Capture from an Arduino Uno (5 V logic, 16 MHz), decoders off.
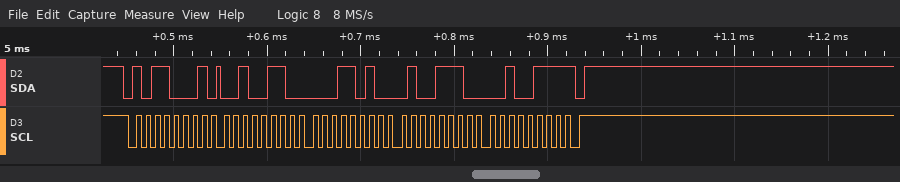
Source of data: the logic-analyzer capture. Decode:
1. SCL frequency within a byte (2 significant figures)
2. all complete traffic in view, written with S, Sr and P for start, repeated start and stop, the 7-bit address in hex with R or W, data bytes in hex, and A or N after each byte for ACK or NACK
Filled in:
100 kHz
S 58R A 26 A 1A A 4E A 27 N P
